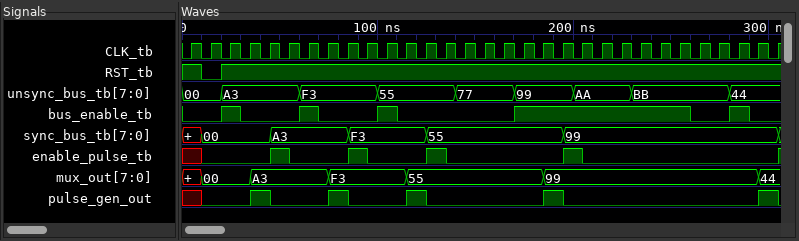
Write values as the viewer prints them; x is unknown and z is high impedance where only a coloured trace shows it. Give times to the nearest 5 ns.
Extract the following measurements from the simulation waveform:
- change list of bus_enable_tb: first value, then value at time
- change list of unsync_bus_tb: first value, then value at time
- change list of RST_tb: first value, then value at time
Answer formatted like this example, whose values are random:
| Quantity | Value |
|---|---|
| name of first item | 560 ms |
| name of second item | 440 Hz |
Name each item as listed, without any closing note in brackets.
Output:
| Quantity | Value |
|---|---|
| change list of bus_enable_tb: first value, then value at time | 0, 1 at 20 ns, 0 at 30 ns, 1 at 60 ns, 0 at 70 ns, 1 at 100 ns, 0 at 110 ns, 1 at 170 ns, 0 at 260 ns, 1 at 280 ns, 0 at 290 ns |
| change list of unsync_bus_tb: first value, then value at time | 00, A3 at 20 ns, F3 at 60 ns, 55 at 100 ns, 77 at 140 ns, 99 at 170 ns, AA at 200 ns, BB at 230 ns, 44 at 280 ns |
| change list of RST_tb: first value, then value at time | 1, 0 at 10 ns, 1 at 20 ns |
